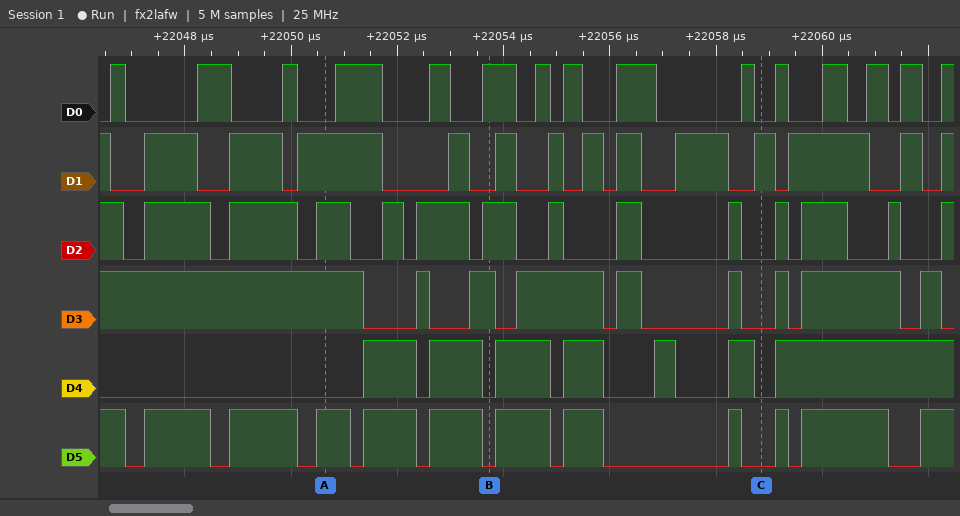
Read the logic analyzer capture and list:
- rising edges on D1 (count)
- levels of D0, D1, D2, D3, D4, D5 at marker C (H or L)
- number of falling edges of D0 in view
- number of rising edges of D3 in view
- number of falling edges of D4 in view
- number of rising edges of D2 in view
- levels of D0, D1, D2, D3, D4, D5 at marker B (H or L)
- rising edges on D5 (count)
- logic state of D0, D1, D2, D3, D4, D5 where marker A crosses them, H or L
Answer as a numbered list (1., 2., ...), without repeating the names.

1. 13
2. D0=L, D1=H, D2=L, D3=L, D4=L, D5=L
3. 14
4. 8
5. 6
6. 13
7. D0=H, D1=L, D2=H, D3=H, D4=L, D5=L
8. 11
9. D0=L, D1=H, D2=H, D3=H, D4=L, D5=H
